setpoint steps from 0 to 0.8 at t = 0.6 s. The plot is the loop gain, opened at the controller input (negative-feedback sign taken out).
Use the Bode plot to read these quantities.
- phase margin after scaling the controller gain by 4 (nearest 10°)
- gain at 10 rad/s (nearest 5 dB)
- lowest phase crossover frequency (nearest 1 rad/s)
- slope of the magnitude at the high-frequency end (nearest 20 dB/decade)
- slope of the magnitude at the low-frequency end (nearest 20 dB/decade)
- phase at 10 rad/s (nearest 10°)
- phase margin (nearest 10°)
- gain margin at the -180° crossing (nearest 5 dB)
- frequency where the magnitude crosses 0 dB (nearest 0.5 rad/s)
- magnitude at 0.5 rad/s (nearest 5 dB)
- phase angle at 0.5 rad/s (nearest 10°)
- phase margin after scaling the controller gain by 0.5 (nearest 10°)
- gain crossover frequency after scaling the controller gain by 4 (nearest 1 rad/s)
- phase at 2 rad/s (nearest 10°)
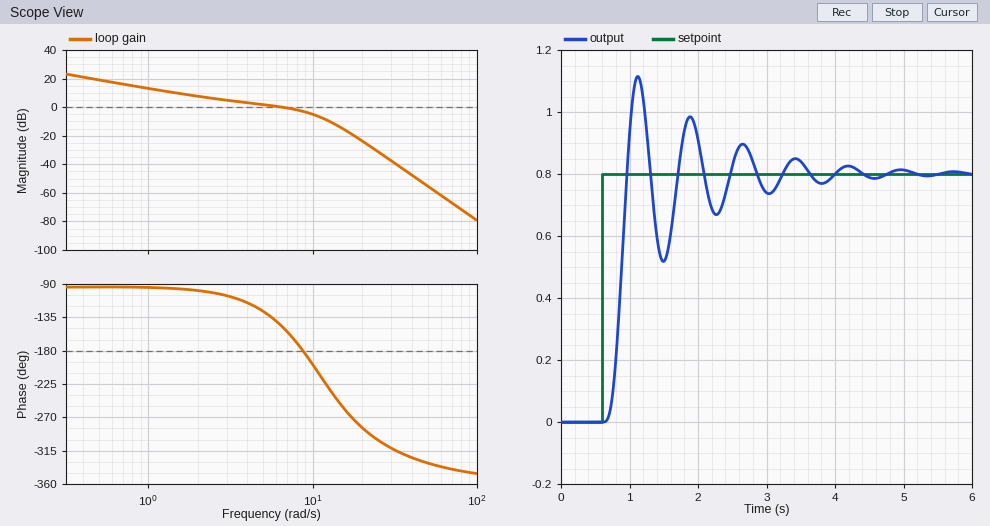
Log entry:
-60°
-5 dB
9 rad/s
-80 dB/decade
-20 dB/decade
-200°
30°
5 dB
6.5 rad/s
20 dB
-90°
80°
14 rad/s
-100°
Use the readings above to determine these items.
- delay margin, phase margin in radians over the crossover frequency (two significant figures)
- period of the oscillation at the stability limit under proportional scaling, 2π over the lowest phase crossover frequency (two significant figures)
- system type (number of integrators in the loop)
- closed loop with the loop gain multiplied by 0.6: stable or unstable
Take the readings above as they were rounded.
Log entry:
0.081 s
0.70 s
1
stable
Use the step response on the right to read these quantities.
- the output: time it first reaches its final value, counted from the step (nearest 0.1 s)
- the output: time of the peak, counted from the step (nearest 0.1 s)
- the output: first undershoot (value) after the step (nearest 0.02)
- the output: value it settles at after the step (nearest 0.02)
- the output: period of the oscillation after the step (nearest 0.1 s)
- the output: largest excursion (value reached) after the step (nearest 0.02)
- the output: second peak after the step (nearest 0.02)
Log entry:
0.4 s
0.5 s
0.52
0.80
0.8 s
1.12
0.98
